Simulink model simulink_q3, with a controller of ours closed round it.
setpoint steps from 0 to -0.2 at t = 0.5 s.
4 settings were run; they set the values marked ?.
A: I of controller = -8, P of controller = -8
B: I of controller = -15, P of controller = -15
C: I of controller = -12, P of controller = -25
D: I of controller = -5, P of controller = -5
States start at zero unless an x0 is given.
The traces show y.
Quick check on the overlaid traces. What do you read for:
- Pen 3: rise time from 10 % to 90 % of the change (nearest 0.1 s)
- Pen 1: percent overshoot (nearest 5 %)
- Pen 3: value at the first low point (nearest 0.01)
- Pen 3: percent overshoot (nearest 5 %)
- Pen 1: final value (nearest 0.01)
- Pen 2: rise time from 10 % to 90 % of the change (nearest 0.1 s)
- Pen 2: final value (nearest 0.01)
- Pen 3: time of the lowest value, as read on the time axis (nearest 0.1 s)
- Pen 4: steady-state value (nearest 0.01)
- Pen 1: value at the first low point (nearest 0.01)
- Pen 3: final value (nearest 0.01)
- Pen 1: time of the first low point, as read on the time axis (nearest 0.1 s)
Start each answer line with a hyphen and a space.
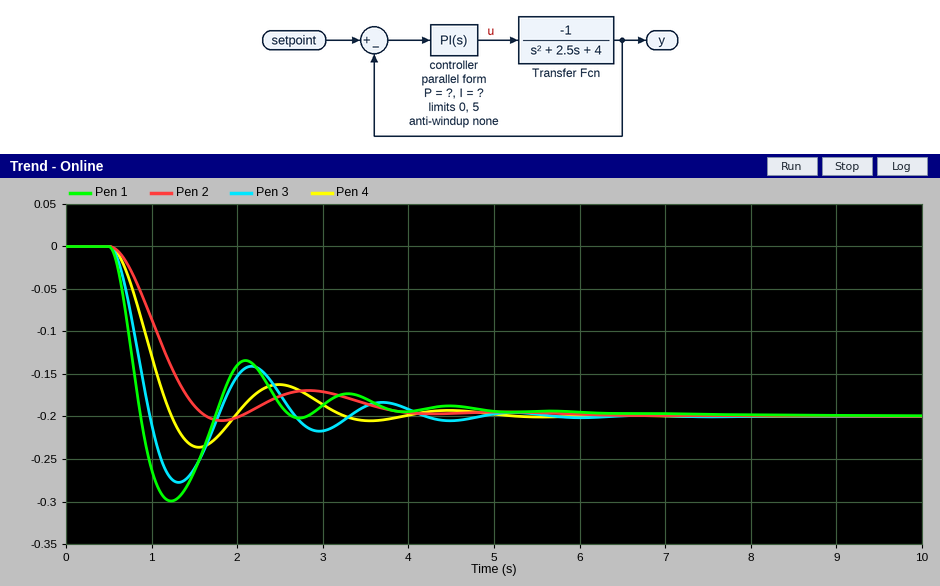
- 0.3 s
- 50 %
- -0.28
- 40 %
- -0.20
- 0.7 s
- -0.20
- 1.3 s
- -0.20
- -0.30
- -0.20
- 1.2 s
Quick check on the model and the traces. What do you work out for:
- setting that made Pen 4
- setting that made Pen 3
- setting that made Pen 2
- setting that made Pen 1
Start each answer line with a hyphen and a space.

- A
- B
- D
- C
